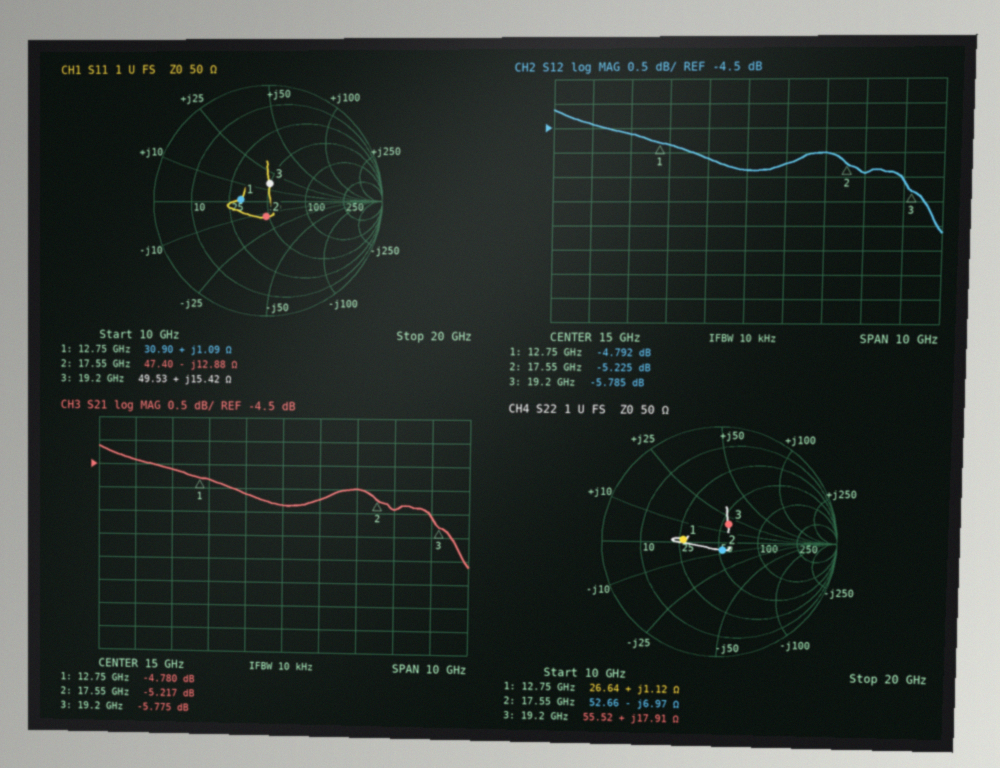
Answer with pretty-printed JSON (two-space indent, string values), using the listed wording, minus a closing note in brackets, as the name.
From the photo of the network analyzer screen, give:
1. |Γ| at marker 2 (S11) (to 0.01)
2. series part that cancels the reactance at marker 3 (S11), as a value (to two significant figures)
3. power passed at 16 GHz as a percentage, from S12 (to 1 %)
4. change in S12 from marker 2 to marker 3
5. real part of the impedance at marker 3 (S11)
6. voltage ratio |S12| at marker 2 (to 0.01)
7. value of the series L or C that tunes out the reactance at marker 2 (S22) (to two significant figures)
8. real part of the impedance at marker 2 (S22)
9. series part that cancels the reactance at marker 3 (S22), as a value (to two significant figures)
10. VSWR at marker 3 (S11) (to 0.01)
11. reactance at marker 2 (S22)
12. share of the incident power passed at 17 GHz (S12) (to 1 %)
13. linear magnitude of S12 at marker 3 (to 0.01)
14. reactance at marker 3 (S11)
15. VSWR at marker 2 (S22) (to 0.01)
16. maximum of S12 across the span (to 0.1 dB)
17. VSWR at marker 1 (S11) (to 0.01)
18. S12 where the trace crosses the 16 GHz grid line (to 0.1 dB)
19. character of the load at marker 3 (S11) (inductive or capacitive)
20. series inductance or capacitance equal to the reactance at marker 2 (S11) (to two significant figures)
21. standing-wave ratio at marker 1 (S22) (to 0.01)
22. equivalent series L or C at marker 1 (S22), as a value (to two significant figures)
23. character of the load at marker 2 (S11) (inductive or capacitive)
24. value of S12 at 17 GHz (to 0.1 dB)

{
  "|Γ| at marker 2 (S11)": "0.13",
  "series part that cancels the reactance at marker 3 (S11), as a value": "540 fF",
  "power passed at 16 GHz as a percentage, from S12": "30 %",
  "change in S12 from marker 2 to marker 3": "-0.560 dB",
  "real part of the impedance at marker 3": "49.53 Ω",
  "voltage ratio |S12| at marker 2": "0.55",
  "value of the series L or C that tunes out the reactance at marker 2 (S22)": "63 pH",
  "real part of the impedance at marker 2": "52.66 Ω",
  "series part that cancels the reactance at marker 3 (S22), as a value": "460 fF",
  "VSWR at marker 3 (S11)": "1.36",
  "reactance at marker 2": "-6.97 Ω",
  "share of the incident power passed at 17 GHz (S12)": "32 %",
  "linear magnitude of S12 at marker 3": "0.51",
  "reactance at marker 3": "+15.42 Ω",
  "VSWR at marker 2 (S22)": "1.16",
  "maximum of S12 across the span": "-4.1 dB",
  "VSWR at marker 1 (S11)": "1.62",
  "S12 where the trace crosses the 16 GHz grid line": "-5.2 dB",
  "character of the load at marker 3 (S11)": "inductive",
  "series inductance or capacitance equal to the reactance at marker 2 (S11)": "700 fF",
  "standing-wave ratio at marker 1 (S22)": "1.88",
  "equivalent series L or C at marker 1 (S22), as a value": "14 pH",
  "character of the load at marker 2 (S11)": "capacitive",
  "value of S12 at 17 GHz": "-5.0 dB"
}
